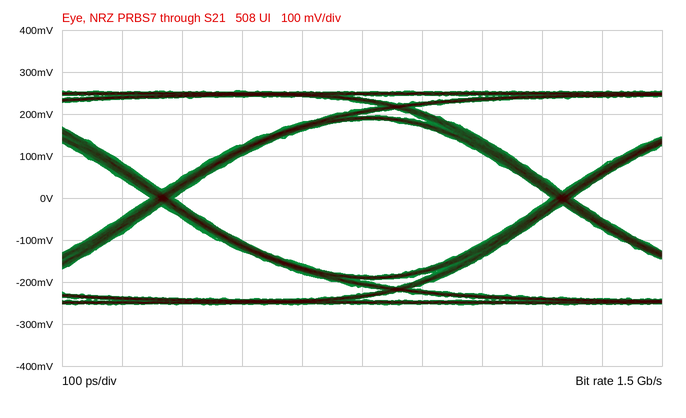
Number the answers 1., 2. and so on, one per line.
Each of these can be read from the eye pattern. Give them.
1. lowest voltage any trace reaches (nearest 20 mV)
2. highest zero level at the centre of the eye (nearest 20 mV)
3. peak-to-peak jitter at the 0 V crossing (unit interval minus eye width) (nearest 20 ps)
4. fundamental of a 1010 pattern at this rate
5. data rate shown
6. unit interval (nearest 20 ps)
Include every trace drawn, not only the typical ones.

1. -260 mV
2. -180 mV
3. 40 ps
4. 750 MHz
5. 1.5 Gb/s
6. 660 ps
